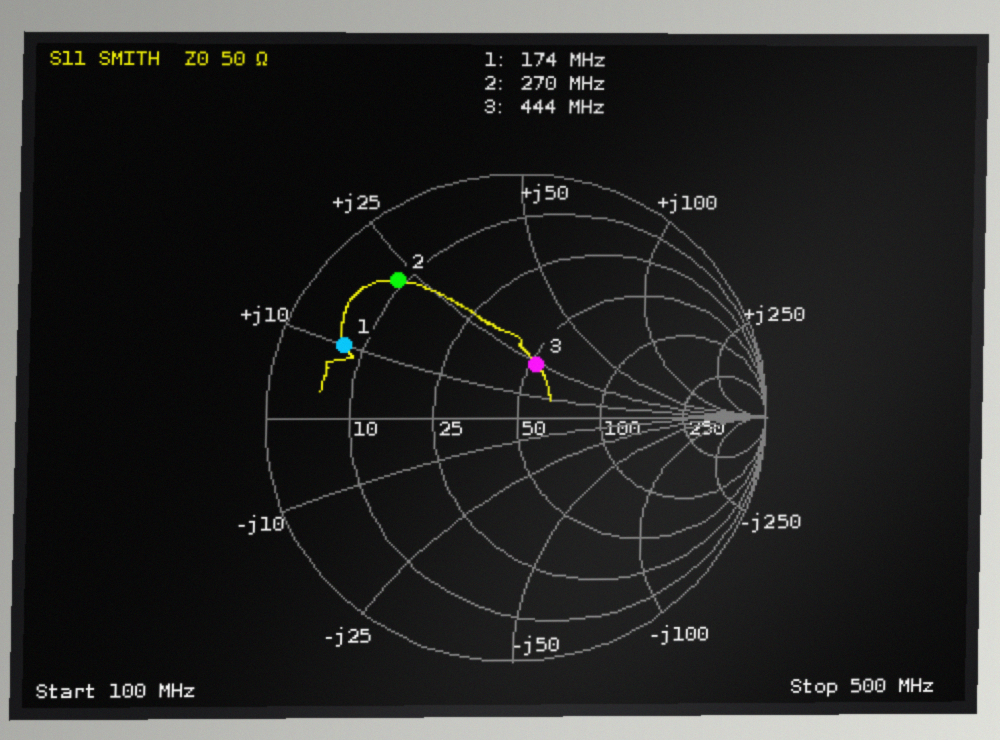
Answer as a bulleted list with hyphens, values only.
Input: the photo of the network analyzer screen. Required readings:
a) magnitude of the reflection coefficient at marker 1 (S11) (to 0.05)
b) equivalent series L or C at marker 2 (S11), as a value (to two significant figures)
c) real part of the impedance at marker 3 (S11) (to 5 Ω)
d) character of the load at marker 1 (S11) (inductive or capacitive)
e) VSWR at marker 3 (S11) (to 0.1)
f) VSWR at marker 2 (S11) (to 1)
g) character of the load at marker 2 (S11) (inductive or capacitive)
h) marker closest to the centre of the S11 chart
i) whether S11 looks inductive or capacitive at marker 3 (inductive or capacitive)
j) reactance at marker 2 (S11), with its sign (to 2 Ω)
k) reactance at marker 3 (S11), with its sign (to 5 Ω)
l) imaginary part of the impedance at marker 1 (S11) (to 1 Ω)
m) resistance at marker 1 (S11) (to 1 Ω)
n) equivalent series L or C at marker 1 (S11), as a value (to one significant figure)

- 0.75
- 13 nH
- 50 Ω
- inductive
- 1.6
- 7
- inductive
- marker 3
- inductive
- +22 Ω
- +25 Ω
- +10 Ω
- 7 Ω
- 9 nH
